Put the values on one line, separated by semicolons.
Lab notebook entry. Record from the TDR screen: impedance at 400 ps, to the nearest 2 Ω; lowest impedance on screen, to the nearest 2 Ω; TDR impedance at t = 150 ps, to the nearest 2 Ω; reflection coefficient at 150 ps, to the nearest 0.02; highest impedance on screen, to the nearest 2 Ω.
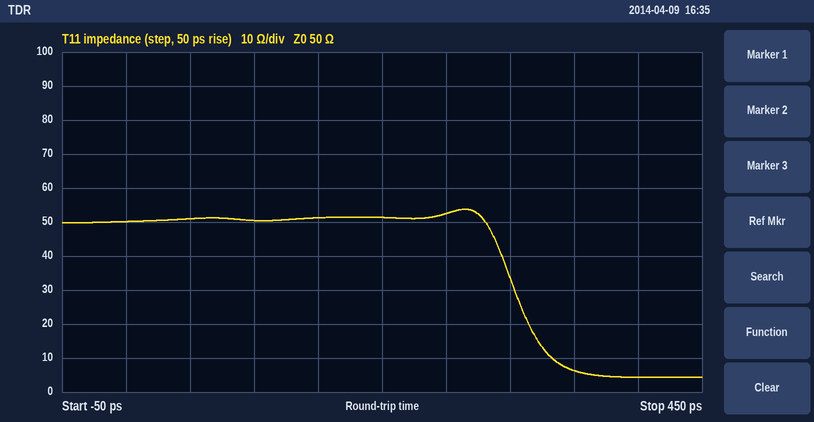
4 Ω; 4 Ω; 52 Ω; +0.02; 54 Ω
